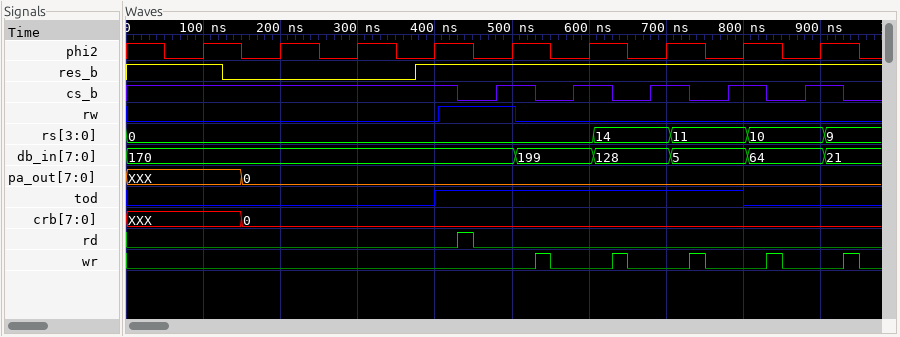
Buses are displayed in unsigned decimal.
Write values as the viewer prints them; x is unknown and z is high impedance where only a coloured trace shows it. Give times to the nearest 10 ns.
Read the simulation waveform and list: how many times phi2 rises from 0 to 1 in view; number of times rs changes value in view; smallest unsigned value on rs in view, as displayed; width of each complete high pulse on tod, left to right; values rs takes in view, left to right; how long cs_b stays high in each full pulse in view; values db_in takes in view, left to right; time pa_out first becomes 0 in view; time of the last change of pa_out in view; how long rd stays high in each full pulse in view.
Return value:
9
4
0
400 ns
0, 14, 11, 10, 9
50 ns, 50 ns, 50 ns, 50 ns, 50 ns
170, 199, 128, 5, 64, 21
150 ns
150 ns
20 ns
